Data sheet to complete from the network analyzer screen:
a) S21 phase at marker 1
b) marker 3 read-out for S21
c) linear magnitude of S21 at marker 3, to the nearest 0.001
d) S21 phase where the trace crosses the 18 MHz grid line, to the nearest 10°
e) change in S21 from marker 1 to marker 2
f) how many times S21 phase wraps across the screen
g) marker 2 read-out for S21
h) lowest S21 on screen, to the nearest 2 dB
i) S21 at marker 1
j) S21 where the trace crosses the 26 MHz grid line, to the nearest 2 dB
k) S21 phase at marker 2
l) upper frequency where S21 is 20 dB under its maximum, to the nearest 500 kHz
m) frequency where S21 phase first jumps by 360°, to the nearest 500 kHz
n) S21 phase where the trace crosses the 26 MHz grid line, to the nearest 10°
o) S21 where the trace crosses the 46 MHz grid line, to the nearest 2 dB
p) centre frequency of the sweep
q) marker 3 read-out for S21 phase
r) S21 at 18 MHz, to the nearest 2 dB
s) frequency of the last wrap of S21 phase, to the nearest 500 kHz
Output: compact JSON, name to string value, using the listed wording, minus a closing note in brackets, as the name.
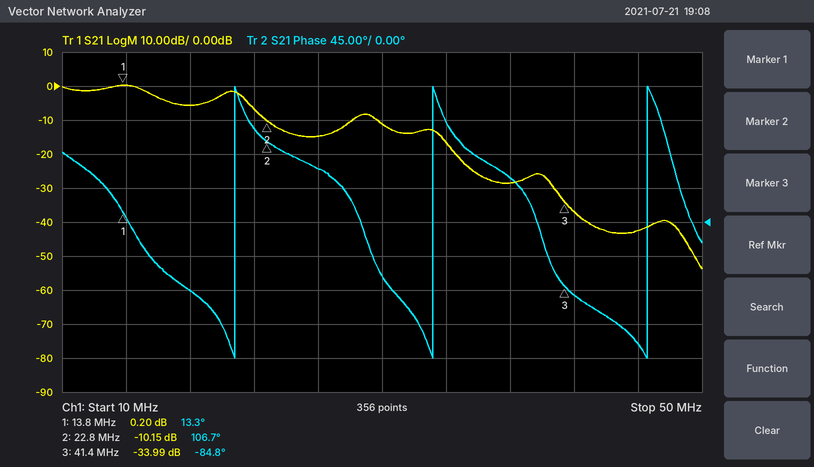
{"S21 phase at marker 1": "13.3°", "marker 3 read-out for S21": "-33.99 dB", "linear magnitude of S21 at marker 3, to the nearest 0.001": "0.020", "S21 phase where the trace crosses the 18 MHz grid line, to the nearest 10°": "-90°", "change in S21 from marker 1 to marker 2": "-10.35 dB", "how many times S21 phase wraps across the screen": "3", "marker 2 read-out for S21": "-10.15 dB", "lowest S21 on screen, to the nearest 2 dB": "-54 dB", "S21 at marker 1": "0.20 dB", "S21 where the trace crosses the 26 MHz grid line, to the nearest 2 dB": "-14 dB", "S21 phase at marker 2": "106.7°", "upper frequency where S21 is 20 dB under its maximum, to the nearest 500 kHz": "34.5 MHz", "frequency where S21 phase first jumps by 360°, to the nearest 500 kHz": "21.0 MHz", "S21 phase where the trace crosses the 26 MHz grid line, to the nearest 10°": "70°", "S21 where the trace crosses the 46 MHz grid line, to the nearest 2 dB": "-42 dB", "centre frequency of the sweep": "30 MHz", "marker 3 read-out for S21 phase": "-84.8°", "S21 at 18 MHz, to the nearest 2 dB": "-6 dB", "frequency of the last wrap of S21 phase, to the nearest 500 kHz": "46.5 MHz"}
